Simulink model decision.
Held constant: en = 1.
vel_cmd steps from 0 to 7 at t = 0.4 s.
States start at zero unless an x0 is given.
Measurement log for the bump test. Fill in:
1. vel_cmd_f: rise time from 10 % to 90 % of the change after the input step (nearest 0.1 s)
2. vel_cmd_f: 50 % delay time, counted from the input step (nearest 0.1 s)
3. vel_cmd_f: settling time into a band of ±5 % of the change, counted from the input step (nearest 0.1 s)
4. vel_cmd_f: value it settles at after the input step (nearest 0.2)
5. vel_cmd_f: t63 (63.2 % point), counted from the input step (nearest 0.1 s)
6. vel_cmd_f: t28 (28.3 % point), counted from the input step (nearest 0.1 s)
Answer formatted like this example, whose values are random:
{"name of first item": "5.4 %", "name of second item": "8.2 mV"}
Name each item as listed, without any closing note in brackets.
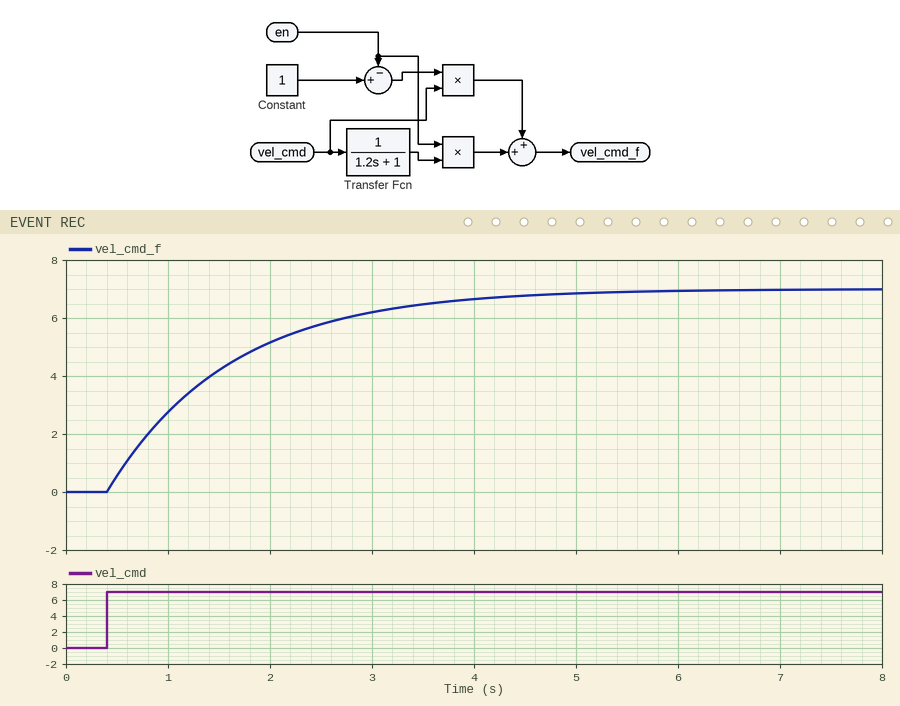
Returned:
{"vel_cmd_f: rise time from 10 % to 90 % of the change after the input step": "2.6 s", "vel_cmd_f: 50 % delay time, counted from the input step": "0.8 s", "vel_cmd_f: settling time into a band of ±5 % of the change, counted from the input step": "3.6 s", "vel_cmd_f: value it settles at after the input step": "7.0", "vel_cmd_f: t63 (63.2 % point), counted from the input step": "1.2 s", "vel_cmd_f: t28 (28.3 % point), counted from the input step": "0.4 s"}
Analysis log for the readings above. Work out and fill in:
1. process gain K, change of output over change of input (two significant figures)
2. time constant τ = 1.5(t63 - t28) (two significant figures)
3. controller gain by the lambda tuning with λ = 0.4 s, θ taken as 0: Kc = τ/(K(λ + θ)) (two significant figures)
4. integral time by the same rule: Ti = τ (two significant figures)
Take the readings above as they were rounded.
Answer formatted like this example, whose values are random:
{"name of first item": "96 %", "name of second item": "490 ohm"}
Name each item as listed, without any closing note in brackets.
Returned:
{"process gain K, change of output over change of input": "1.0", "time constant τ = 1.5(t63 - t28)": "1.2 s", "controller gain by the lambda tuning with λ = 0.4 s, θ taken as 0: Kc = τ/(K(λ + θ))": "3.0", "integral time by the same rule: Ti = τ": "1.2 s"}
